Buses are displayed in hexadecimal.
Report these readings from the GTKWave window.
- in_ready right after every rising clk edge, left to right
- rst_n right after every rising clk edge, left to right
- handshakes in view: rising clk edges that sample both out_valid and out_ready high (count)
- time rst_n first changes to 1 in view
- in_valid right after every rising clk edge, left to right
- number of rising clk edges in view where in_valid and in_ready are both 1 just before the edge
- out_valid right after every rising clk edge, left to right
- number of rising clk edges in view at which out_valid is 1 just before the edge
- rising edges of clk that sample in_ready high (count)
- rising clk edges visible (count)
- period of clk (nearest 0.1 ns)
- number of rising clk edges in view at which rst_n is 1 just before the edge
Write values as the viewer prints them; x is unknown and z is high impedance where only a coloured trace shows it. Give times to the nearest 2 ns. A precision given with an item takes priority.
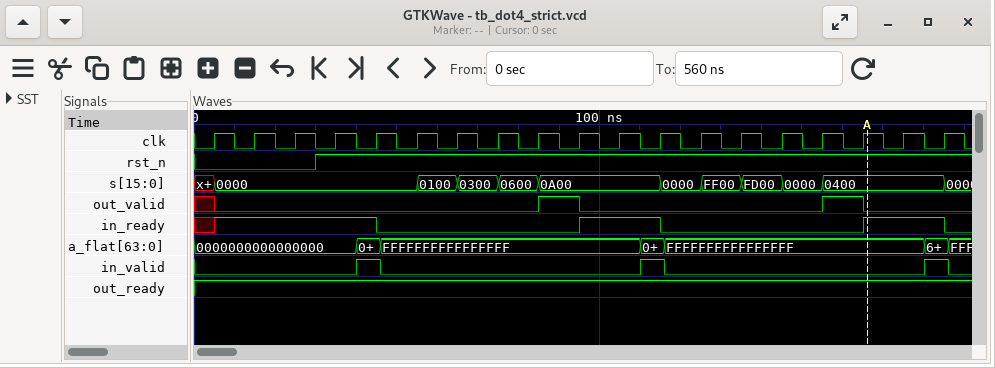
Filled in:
1 1 1 1 0 0 0 0 0 1 1 0 0 0 0 0 1 1 0
0 0 0 1 1 1 1 1 1 1 1 1 1 1 1 1 1 1 1
2
30 ns
0 0 0 0 1 0 0 0 0 0 0 1 0 0 0 0 0 0 1
3
0 0 0 0 0 0 0 0 1 0 0 0 0 0 0 1 0 0 0
2
8
19
10 ns
16
